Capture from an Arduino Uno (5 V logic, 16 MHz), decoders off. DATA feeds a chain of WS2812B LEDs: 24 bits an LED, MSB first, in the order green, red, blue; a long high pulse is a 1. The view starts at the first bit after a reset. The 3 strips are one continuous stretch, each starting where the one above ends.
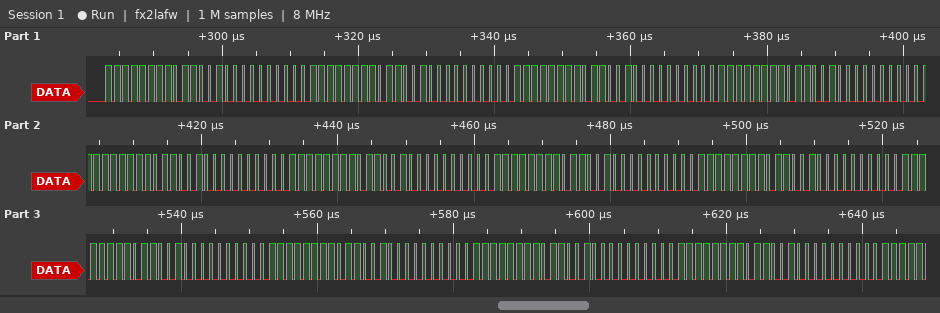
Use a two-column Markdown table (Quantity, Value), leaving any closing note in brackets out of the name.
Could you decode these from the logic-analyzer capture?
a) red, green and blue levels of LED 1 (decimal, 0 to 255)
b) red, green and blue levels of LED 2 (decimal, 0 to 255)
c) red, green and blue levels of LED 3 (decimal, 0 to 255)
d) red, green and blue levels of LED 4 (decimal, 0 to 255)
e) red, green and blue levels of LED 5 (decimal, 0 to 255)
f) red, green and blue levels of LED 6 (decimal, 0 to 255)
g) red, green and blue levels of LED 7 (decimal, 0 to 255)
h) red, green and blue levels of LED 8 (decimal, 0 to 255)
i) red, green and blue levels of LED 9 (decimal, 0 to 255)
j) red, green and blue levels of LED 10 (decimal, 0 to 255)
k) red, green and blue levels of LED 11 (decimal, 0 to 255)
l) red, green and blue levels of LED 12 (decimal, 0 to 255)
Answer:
| Quantity | Value |
|---|---|
| red, green and blue levels of LED 1 | 100, 255, 0 |
| red, green and blue levels of LED 2 | 100, 255, 0 |
| red, green and blue levels of LED 3 | 100, 255, 0 |
| red, green and blue levels of LED 4 | 100, 255, 0 |
| red, green and blue levels of LED 5 | 100, 255, 0 |
| red, green and blue levels of LED 6 | 100, 255, 0 |
| red, green and blue levels of LED 7 | 100, 255, 0 |
| red, green and blue levels of LED 8 | 100, 255, 0 |
| red, green and blue levels of LED 9 | 100, 255, 0 |
| red, green and blue levels of LED 10 | 100, 255, 0 |
| red, green and blue levels of LED 11 | 100, 255, 0 |
| red, green and blue levels of LED 12 | 100, 255, 0 |
